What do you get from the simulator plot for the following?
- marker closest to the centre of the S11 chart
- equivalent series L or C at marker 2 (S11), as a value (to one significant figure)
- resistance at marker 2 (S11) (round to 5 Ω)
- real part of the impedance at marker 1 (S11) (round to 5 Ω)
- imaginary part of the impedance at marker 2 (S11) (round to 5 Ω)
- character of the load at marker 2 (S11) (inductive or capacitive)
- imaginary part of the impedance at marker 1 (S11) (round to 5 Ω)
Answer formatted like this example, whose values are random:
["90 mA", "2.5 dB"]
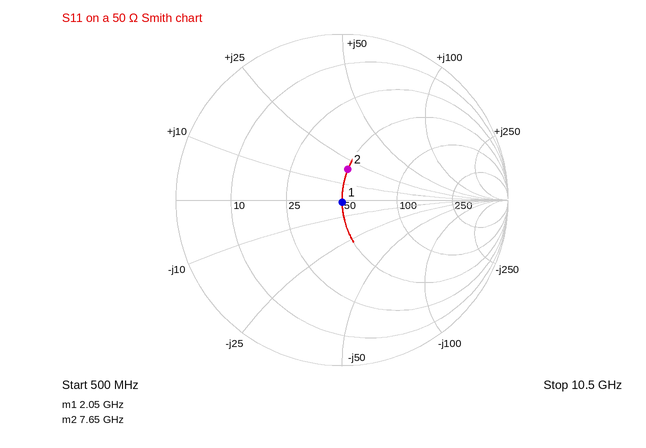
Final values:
["marker 1", "400 pH", "50 Ω", "50 Ω", "+20 Ω", "inductive", "0 Ω"]
